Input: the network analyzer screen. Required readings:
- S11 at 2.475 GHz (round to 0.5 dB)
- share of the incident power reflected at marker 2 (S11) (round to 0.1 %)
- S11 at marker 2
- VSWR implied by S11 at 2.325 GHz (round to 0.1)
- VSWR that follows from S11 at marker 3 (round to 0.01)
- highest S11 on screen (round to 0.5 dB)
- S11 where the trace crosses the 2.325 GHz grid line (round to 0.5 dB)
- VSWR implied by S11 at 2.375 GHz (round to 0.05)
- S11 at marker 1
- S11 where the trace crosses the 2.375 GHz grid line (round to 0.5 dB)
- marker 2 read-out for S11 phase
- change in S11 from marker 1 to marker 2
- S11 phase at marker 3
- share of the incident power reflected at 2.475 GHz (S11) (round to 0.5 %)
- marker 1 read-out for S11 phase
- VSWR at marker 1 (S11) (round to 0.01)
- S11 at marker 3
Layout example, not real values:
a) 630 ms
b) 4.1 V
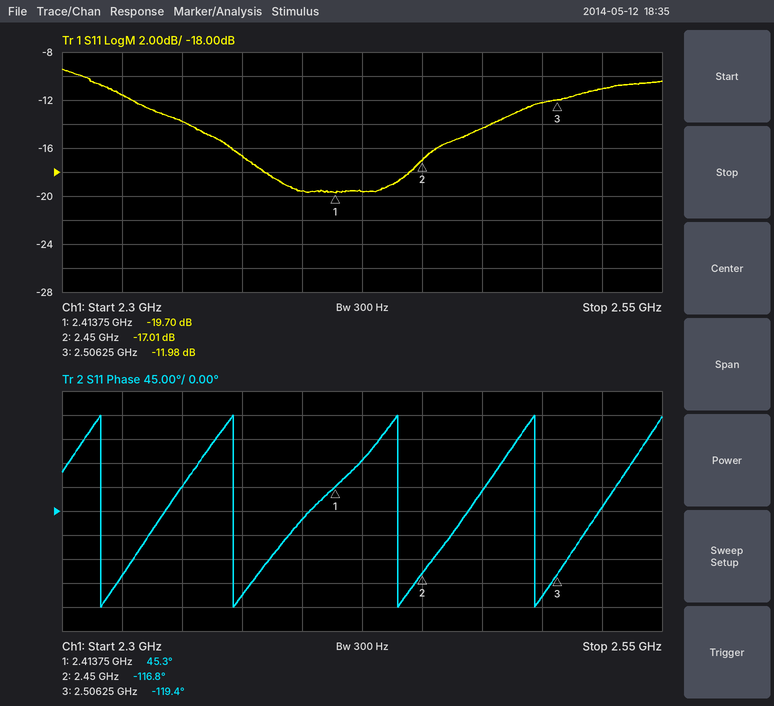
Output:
a) -14.5 dB
b) 2.0 %
c) -17.01 dB
d) 1.7
e) 1.67
f) -9.5 dB
g) -11.5 dB
h) 1.35
i) -19.70 dB
j) -16.5 dB
k) -116.8°
l) 2.69 dB
m) -119.4°
n) 3.5 %
o) 45.3°
p) 1.23
q) -11.98 dB
